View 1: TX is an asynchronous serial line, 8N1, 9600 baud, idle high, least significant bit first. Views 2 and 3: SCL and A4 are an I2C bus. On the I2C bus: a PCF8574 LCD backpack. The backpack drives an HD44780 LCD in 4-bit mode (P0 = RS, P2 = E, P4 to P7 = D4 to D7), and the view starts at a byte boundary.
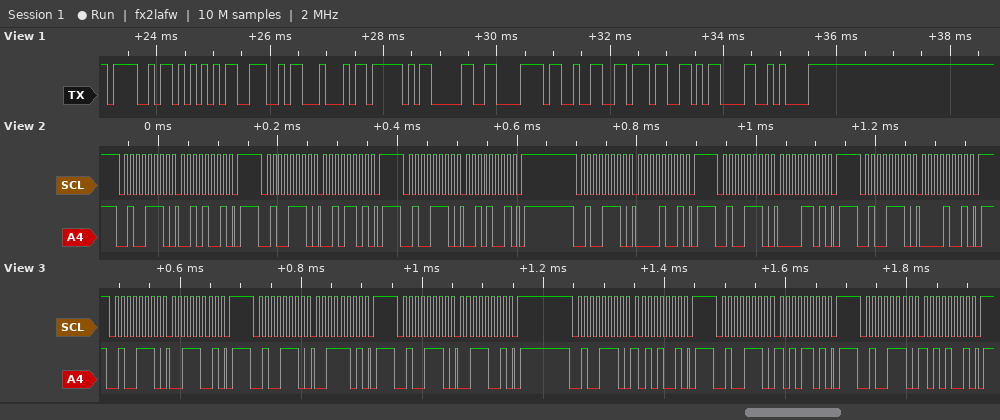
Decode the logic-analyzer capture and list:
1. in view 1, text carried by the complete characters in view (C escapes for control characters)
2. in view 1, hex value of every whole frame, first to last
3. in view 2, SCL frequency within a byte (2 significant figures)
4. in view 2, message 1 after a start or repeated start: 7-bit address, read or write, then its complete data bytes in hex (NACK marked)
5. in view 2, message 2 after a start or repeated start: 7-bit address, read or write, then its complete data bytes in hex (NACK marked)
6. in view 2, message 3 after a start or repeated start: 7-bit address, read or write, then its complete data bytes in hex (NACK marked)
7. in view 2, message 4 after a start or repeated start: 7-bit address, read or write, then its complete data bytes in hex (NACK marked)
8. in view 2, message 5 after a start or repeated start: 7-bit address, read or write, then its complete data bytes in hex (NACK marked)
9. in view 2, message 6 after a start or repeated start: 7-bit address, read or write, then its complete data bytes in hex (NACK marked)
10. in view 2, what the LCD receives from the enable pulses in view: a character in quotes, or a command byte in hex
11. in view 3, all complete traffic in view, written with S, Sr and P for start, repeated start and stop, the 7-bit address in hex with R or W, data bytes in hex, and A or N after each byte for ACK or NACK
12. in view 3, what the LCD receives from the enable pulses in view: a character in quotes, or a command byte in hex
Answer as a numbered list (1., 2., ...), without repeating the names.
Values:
1. "OUND_0x27\r\n"
2. 4F 55 4E 44 5F 30 78 32 37 0D 0A
3. 100 kHz
4. 0x27 write: 29
5. 0x27 write: 2D
6. 0x27 write: 29
7. 0x27 write: 09
8. 0x27 write: 0D
9. 0x27 write: 09
10. ' '
11. S 27W A 39 A P S 27W A 3D A P S 27W A 39 A P S 27W A A9 A P S 27W A AD A P S 27W A A9 A P
12. ':'
